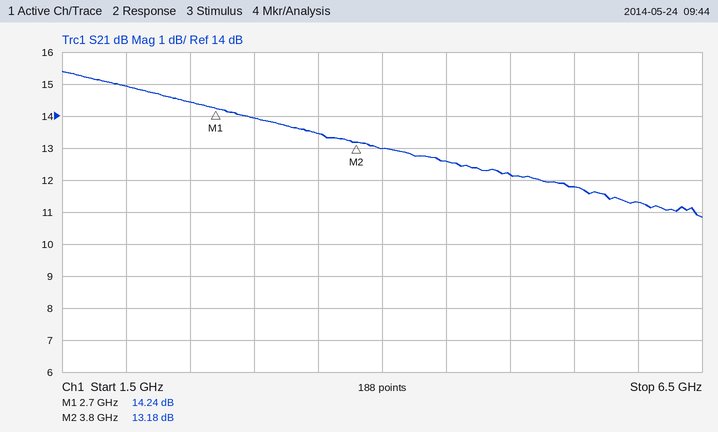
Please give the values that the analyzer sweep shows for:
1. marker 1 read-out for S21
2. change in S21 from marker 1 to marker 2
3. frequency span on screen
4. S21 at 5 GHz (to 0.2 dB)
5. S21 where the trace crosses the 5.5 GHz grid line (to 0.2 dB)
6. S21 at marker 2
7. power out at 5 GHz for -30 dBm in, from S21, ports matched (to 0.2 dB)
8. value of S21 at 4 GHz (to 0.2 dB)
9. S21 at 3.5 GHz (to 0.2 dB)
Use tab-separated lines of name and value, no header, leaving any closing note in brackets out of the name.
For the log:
marker 1 read-out for S21	14.24 dB
change in S21 from marker 1 to marker 2	-1.06 dB
frequency span on screen	5 GHz
S21 at 5 GHz	12.2 dB
S21 where the trace crosses the 5.5 GHz grid line	11.8 dB
S21 at marker 2	13.18 dB
power out at 5 GHz for -30 dBm in, from S21, ports matched	-17.8 dBm
value of S21 at 4 GHz	13.0 dB
S21 at 3.5 GHz	13.4 dB
